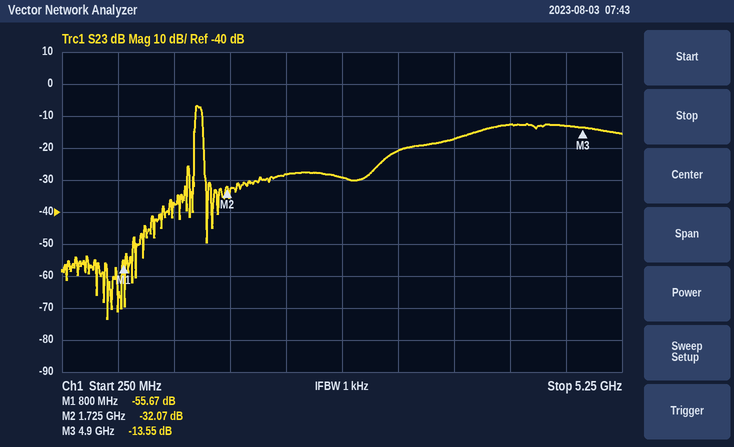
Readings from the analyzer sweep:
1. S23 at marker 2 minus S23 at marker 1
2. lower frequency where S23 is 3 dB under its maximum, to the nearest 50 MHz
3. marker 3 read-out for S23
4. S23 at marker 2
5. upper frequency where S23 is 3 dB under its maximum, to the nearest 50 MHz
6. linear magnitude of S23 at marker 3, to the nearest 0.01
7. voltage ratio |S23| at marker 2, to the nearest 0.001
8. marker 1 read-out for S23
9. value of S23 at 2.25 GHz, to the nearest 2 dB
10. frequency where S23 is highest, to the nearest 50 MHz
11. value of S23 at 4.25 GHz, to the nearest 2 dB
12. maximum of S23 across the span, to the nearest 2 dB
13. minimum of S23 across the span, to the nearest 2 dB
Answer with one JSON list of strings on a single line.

["23.60 dB", "1.45 GHz", "-13.55 dB", "-32.07 dB", "1.50 GHz", "0.21", "0.025", "-55.67 dB", "-28 dB", "1.45 GHz", "-12 dB", "-6 dB", "-74 dB"]
